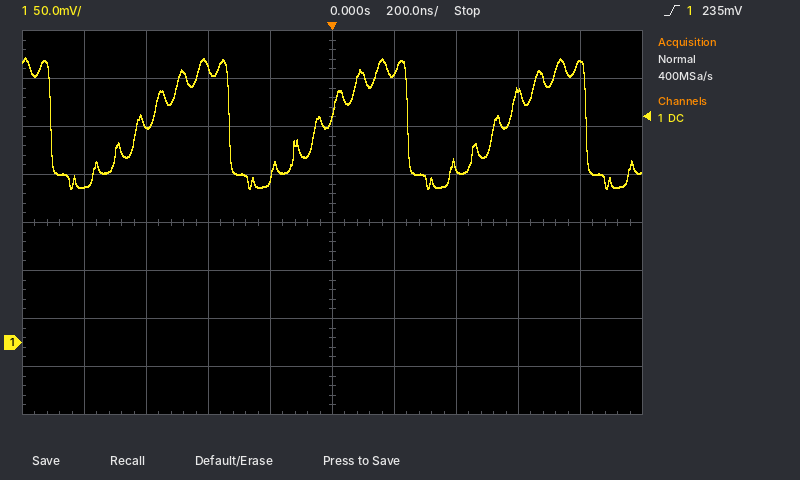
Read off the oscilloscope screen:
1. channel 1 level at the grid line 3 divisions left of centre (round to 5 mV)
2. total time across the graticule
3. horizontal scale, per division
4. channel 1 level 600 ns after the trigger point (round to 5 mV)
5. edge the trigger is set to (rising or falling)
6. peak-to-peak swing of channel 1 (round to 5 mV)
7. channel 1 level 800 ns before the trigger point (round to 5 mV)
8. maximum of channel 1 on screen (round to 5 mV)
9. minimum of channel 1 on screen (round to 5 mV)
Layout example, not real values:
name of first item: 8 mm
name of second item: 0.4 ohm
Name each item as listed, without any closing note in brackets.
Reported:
channel 1 level at the grid line 3 divisions left of centre: 225 mV
total time across the graticule: 2 µs
horizontal scale, per division: 200 ns
channel 1 level 600 ns after the trigger point: 260 mV
edge the trigger is set to: rising
peak-to-peak swing of channel 1: 135 mV
channel 1 level 800 ns before the trigger point: 160 mV
maximum of channel 1 on screen: 295 mV
minimum of channel 1 on screen: 160 mV
